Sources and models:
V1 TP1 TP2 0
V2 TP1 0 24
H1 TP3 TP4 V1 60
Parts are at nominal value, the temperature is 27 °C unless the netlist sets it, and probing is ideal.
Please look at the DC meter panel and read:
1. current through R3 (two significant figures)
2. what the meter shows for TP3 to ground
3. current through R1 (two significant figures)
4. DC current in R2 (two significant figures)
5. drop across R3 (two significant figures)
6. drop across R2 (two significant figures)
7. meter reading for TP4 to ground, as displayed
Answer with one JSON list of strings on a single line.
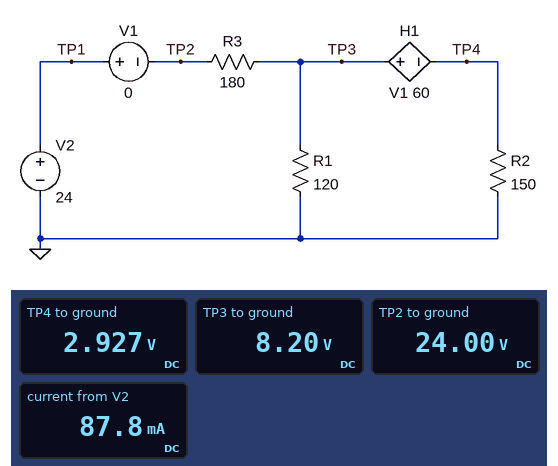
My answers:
["88 mA", "8.20 V", "68 mA", "20 mA", "16 V", "2.9 V", "2.927 V"]
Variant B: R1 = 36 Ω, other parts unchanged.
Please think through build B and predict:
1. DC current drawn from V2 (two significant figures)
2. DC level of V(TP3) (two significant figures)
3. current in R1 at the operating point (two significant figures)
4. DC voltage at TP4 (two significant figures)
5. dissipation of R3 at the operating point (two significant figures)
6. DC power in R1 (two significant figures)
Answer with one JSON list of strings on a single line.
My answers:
["110 mA", "4.4 V", "120 mA", "-2.1 V", "2.1 W", "540 mW"]
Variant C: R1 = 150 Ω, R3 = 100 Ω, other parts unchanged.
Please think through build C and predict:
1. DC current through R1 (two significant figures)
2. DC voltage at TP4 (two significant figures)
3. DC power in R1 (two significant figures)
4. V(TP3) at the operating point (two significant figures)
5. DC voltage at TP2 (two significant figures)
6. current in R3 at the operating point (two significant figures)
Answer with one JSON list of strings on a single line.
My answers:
["82 mA", "5.3 V", "1.0 W", "12 V", "24 V", "120 mA"]
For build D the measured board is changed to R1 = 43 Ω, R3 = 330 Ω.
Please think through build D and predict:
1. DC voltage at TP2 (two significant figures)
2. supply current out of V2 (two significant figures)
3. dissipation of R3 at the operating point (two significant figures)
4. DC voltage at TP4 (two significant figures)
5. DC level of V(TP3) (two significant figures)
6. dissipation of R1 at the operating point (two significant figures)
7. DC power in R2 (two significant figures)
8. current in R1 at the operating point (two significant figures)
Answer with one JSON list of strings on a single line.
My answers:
["24 V", "64 mA", "1.3 W", "-840 mV", "3.0 V", "210 mW", "4.7 mW", "69 mA"]
